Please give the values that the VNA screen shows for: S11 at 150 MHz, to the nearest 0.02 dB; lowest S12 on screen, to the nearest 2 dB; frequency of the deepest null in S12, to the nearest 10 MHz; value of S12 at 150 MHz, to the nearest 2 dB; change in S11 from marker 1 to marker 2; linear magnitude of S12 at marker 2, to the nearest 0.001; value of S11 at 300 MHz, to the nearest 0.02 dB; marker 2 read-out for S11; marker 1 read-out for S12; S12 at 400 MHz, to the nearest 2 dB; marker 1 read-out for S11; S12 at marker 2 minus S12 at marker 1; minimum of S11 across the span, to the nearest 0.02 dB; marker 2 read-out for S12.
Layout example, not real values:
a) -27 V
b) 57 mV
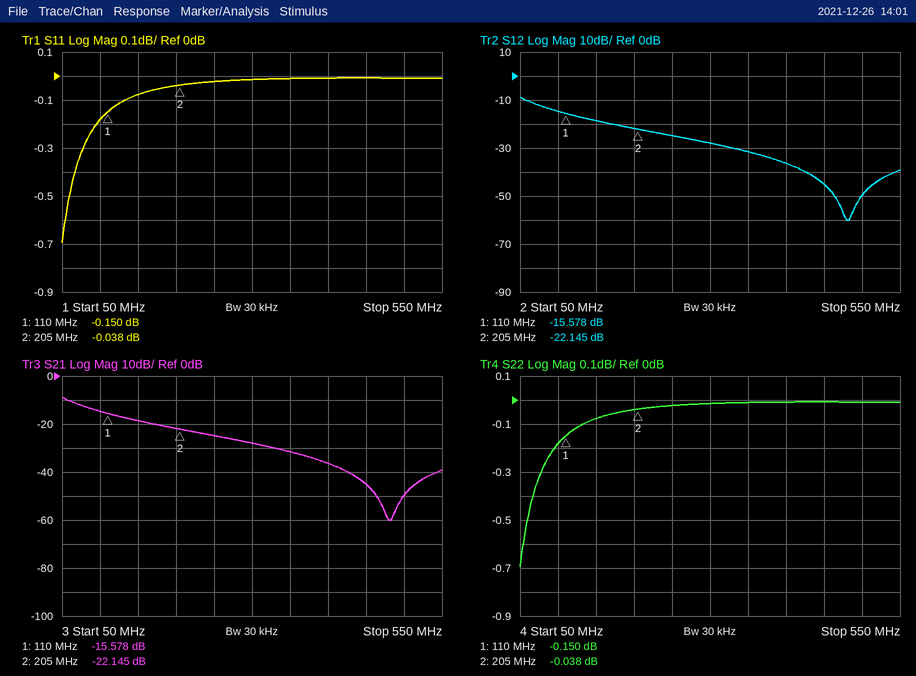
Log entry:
a) -0.08 dB
b) -60 dB
c) 480 MHz
d) -18 dB
e) 0.112 dB
f) 0.078
g) -0.02 dB
h) -0.038 dB
i) -15.578 dB
j) -36 dB
k) -0.150 dB
l) -6.567 dB
m) -0.70 dB
n) -22.145 dB
